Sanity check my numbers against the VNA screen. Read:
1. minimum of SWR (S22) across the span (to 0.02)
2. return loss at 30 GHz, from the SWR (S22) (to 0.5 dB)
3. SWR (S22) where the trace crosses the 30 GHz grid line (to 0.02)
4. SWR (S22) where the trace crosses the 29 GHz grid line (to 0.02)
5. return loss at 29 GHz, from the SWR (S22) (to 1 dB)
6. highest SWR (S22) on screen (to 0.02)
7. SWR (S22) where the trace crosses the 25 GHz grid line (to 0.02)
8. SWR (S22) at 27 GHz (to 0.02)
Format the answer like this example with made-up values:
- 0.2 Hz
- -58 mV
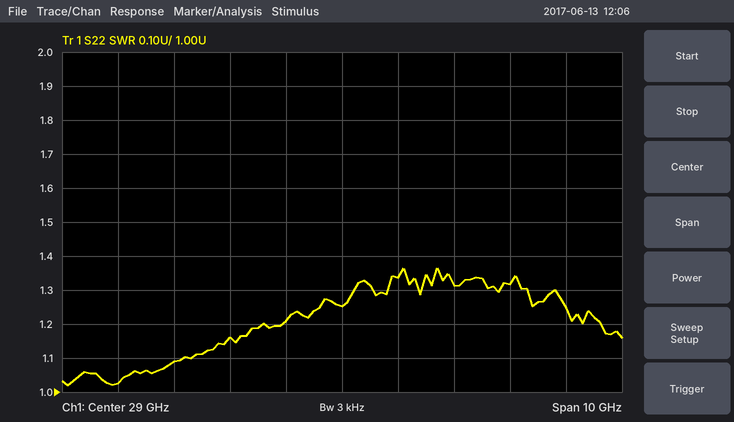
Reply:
- 1.02
- 17.0 dB
- 1.34
- 1.26
- 19 dB
- 1.36
- 1.02
- 1.16
